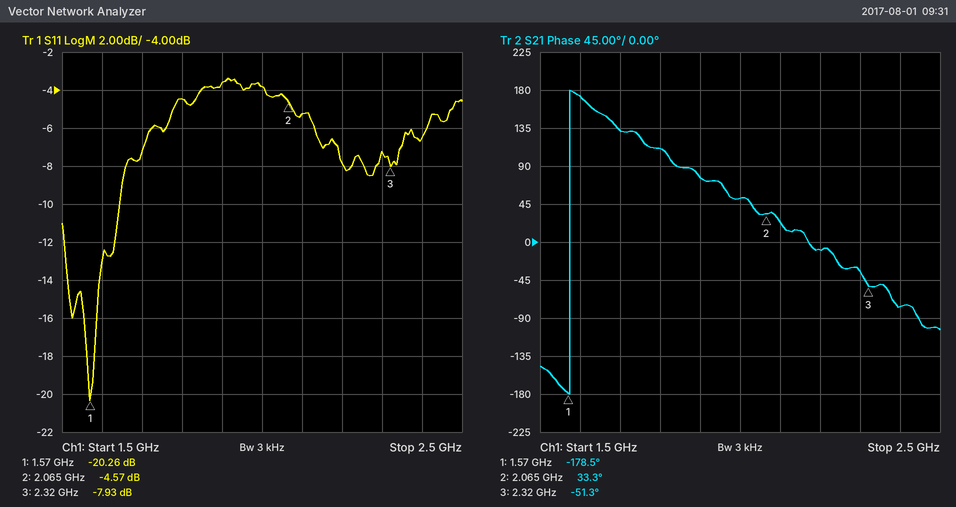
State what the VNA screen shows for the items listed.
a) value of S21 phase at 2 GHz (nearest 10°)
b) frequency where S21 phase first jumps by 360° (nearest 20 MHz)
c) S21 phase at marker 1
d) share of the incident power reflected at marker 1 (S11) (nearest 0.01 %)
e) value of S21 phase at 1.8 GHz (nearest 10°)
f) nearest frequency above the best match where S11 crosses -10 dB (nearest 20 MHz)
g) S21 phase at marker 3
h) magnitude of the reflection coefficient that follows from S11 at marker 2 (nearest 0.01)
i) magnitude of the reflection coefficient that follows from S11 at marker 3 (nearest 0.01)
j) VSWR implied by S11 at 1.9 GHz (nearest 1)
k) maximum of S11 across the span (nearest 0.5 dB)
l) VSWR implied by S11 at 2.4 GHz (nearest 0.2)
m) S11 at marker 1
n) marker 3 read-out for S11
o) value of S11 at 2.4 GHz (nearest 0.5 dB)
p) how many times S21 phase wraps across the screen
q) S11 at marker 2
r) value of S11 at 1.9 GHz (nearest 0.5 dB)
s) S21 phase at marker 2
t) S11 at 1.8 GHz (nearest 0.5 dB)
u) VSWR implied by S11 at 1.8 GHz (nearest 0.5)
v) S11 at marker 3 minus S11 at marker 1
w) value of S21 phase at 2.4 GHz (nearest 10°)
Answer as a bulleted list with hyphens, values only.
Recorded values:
- 50°
- 1.58 GHz
- -178.5°
- 0.94 %
- 110°
- 1.64 GHz
- -51.3°
- 0.59
- 0.40
- 5
- -3.5 dB
- 2.8
- -20.26 dB
- -7.93 dB
- -6.5 dB
- 1
- -4.57 dB
- -3.5 dB
- 33.3°
- -4.5 dB
- 4.0
- 12.33 dB
- -80°
